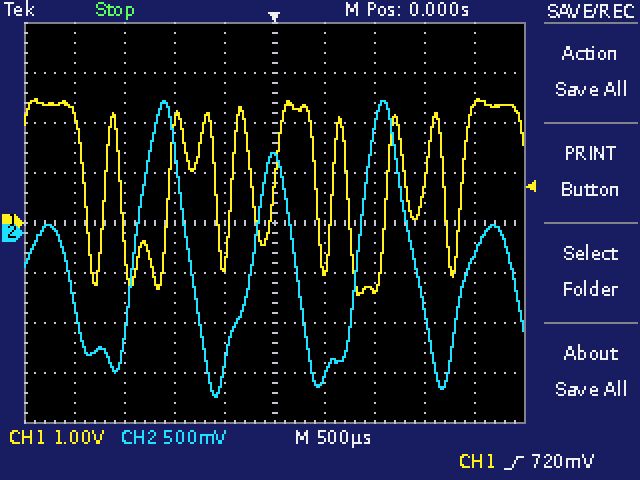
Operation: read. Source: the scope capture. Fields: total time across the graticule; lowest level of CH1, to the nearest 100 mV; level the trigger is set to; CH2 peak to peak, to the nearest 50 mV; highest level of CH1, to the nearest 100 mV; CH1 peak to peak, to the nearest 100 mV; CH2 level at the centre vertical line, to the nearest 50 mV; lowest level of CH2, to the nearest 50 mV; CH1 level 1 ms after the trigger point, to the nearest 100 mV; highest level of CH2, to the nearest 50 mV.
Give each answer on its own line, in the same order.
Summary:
5 ms
-1.4 V
720 mV
2.95 V
2.5 V
3.9 V
750 mV
-1.65 V
-1.3 V
1.30 V
